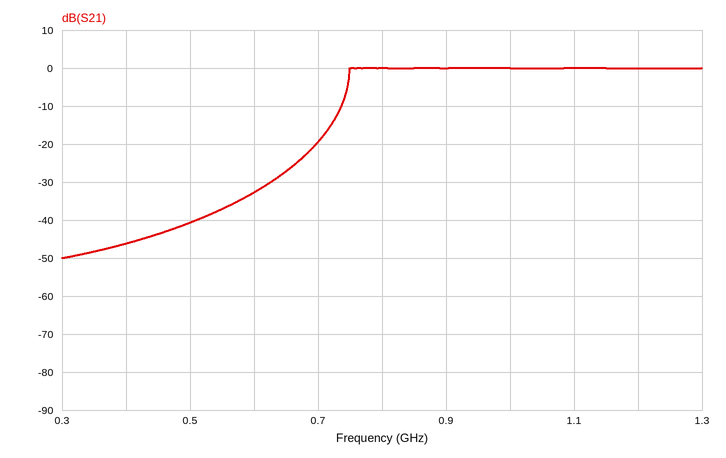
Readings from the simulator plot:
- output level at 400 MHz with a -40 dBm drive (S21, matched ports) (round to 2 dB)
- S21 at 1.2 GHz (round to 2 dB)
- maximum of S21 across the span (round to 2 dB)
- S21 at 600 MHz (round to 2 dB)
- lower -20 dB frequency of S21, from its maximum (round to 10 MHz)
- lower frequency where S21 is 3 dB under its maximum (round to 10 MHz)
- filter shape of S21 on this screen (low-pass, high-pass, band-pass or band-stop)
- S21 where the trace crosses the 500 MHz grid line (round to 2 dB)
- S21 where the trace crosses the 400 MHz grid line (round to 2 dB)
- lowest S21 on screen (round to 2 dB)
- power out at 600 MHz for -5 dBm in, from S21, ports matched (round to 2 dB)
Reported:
-86 dBm
0 dB
0 dB
-32 dB
700 MHz
750 MHz
high-pass
-40 dB
-46 dB
-50 dB
-38 dBm
